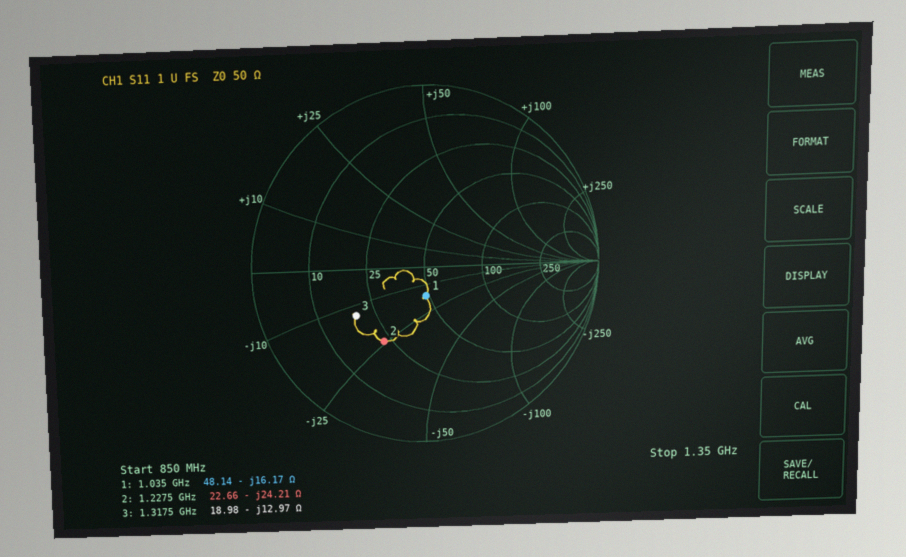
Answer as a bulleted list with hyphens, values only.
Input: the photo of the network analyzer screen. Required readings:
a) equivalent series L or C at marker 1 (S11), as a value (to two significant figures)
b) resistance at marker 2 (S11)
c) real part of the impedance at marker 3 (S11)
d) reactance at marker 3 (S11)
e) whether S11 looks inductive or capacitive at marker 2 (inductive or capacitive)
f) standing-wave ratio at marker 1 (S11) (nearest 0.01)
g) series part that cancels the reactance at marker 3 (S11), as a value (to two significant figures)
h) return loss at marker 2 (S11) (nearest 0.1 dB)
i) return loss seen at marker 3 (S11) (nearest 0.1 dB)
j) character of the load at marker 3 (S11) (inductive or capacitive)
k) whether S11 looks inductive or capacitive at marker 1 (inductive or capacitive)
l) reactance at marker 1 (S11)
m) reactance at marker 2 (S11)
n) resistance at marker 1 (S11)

- 9.5 pF
- 22.66 Ω
- 18.98 Ω
- -12.97 Ω
- capacitive
- 1.39
- 1.6 nH
- 6.4 dB
- 6.4 dB
- capacitive
- capacitive
- -16.17 Ω
- -24.21 Ω
- 48.14 Ω
